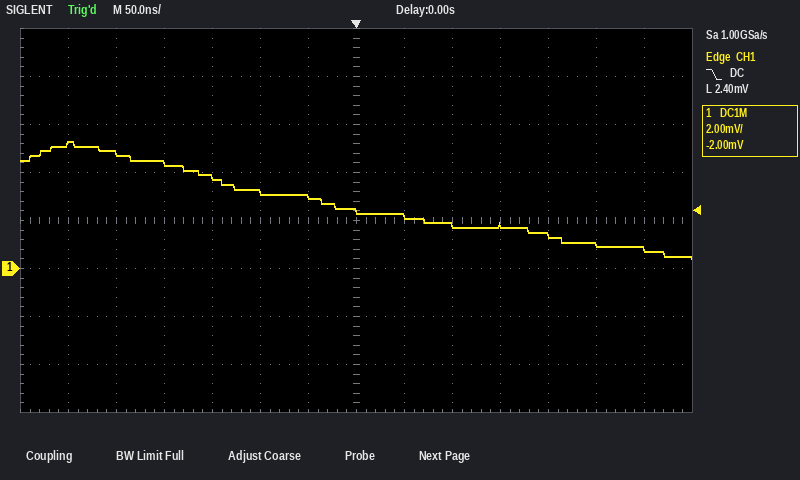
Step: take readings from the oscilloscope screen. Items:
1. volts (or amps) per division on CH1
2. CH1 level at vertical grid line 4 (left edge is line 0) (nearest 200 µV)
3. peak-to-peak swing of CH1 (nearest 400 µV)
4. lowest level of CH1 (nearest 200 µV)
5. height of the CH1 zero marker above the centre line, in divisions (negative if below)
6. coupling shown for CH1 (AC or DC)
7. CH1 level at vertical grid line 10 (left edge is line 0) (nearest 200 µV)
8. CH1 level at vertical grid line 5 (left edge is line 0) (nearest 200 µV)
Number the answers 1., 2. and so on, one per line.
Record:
1. 2 mV
2. 3.8 mV
3. 4.8 mV
4. 400 µV
5. -1.0 div
6. DC
7. 1.8 mV
8. 3.2 mV
